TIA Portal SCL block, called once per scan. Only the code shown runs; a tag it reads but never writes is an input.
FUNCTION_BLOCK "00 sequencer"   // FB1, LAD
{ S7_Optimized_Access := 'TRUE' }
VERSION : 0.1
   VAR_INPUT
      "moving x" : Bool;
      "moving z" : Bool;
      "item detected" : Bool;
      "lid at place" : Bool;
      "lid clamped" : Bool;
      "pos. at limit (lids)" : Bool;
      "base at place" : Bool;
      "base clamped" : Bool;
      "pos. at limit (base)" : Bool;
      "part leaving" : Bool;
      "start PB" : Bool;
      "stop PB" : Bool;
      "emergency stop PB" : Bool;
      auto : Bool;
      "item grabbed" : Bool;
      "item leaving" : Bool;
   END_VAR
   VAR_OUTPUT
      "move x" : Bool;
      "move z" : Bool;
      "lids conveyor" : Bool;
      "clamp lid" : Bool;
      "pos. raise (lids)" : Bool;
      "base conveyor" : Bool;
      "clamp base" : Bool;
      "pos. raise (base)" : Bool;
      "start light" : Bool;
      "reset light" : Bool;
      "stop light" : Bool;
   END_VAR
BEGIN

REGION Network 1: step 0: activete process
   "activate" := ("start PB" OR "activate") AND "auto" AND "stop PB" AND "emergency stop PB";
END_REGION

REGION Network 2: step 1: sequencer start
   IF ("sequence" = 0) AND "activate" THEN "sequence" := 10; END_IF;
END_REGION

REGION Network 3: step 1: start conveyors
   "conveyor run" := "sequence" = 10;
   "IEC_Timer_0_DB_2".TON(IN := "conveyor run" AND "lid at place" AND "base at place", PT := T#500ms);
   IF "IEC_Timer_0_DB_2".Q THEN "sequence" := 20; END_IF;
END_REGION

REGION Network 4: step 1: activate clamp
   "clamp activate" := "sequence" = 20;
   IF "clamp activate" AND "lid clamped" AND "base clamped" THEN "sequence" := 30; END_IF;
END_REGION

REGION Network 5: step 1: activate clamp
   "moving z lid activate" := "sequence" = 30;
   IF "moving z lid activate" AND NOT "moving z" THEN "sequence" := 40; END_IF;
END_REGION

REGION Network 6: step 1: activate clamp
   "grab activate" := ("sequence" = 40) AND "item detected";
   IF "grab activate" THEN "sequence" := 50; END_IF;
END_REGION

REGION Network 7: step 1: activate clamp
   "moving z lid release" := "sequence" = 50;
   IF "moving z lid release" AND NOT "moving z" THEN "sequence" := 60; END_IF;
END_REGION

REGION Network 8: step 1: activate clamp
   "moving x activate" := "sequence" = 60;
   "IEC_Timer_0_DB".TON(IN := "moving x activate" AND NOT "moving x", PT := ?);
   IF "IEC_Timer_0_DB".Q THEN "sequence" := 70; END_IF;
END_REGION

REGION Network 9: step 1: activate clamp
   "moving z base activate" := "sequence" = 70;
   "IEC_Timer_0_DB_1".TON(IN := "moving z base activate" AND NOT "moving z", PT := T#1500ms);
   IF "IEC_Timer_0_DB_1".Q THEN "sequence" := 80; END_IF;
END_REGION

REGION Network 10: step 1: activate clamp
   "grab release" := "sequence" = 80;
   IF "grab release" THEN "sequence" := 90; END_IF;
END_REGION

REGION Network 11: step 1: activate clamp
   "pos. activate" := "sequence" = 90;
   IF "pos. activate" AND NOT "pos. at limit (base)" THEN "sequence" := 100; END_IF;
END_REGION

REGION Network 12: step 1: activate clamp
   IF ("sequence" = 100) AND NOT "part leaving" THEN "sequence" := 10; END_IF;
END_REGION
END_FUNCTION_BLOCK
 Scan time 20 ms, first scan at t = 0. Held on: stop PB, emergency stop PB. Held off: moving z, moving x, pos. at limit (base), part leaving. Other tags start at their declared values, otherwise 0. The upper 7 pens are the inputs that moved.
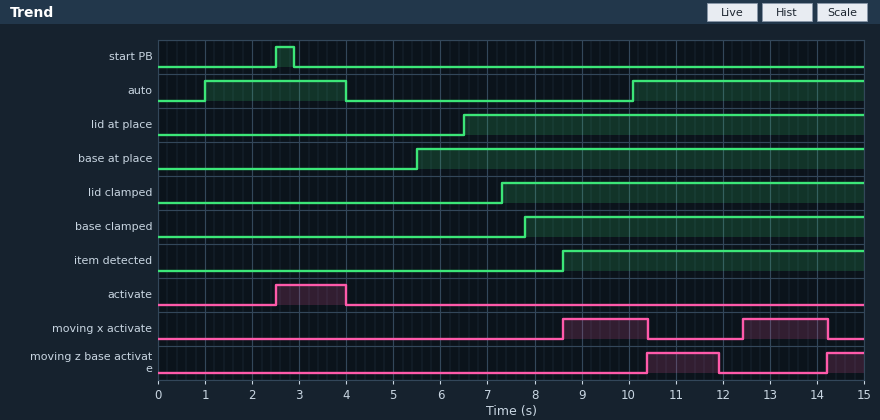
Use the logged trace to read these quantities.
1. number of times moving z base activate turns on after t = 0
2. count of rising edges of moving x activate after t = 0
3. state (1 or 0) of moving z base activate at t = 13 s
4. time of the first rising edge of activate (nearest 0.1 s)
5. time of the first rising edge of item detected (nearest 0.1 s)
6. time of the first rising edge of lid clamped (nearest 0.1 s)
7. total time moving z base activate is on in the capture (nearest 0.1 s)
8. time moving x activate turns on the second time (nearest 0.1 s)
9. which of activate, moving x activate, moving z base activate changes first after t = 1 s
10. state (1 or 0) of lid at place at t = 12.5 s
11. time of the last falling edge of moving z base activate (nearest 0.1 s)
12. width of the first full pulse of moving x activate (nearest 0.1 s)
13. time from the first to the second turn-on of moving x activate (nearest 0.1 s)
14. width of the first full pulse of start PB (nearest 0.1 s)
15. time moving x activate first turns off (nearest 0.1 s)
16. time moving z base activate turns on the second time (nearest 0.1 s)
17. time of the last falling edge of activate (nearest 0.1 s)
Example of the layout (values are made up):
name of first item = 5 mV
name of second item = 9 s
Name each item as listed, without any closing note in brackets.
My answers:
number of times moving z base activate turns on after t = 0 = 2
count of rising edges of moving x activate after t = 0 = 2
state (1 or 0) of moving z base activate at t = 13 s = 0
time of the first rising edge of activate = 2.5 s
time of the first rising edge of item detected = 8.6 s
time of the first rising edge of lid clamped = 7.3 s
total time moving z base activate is on in the capture = 2.3 s
time moving x activate turns on the second time = 12.4 s
which of activate, moving x activate, moving z base activate changes first after t = 1 s = activate
state (1 or 0) of lid at place at t = 12.5 s = 1
time of the last falling edge of moving z base activate = 11.9 s
width of the first full pulse of moving x activate = 1.8 s
time from the first to the second turn-on of moving x activate = 3.8 s
width of the first full pulse of start PB = 0.4 s
time moving x activate first turns off = 10.4 s
time moving z base activate turns on the second time = 14.2 s
time of the last falling edge of activate = 4.0 s
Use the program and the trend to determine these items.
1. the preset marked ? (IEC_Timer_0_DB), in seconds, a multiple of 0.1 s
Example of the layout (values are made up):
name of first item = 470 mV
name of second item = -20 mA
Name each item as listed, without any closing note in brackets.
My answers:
the preset marked ? (IEC_Timer_0_DB), in seconds, a multiple of 0.1 s = 1.8 s
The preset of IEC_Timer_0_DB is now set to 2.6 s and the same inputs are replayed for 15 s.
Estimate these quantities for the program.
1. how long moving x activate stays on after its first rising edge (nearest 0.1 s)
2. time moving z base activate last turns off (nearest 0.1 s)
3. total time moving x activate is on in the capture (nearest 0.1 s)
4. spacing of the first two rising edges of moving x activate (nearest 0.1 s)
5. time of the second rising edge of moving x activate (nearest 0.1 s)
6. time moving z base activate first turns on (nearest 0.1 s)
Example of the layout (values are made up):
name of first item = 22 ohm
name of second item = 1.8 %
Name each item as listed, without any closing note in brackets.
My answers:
how long moving x activate stays on after its first rising edge = 2.6 s
time moving z base activate last turns off = 12.7 s
total time moving x activate is on in the capture = 4.4 s
spacing of the first two rising edges of moving x activate = 4.6 s
time of the second rising edge of moving x activate = 13.2 s
time moving z base activate first turns on = 11.2 s
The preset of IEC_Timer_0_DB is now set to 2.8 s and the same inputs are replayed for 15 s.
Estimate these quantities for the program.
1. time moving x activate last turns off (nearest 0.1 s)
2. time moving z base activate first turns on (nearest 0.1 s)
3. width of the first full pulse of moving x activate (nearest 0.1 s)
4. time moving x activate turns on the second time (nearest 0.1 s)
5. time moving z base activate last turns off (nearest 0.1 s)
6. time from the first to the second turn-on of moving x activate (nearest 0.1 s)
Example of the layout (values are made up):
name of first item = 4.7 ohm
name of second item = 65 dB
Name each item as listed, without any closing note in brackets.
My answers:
time moving x activate last turns off = 11.4 s
time moving z base activate first turns on = 11.4 s
width of the first full pulse of moving x activate = 2.8 s
time moving x activate turns on the second time = 13.4 s
time moving z base activate last turns off = 12.9 s
time from the first to the second turn-on of moving x activate = 4.8 s
